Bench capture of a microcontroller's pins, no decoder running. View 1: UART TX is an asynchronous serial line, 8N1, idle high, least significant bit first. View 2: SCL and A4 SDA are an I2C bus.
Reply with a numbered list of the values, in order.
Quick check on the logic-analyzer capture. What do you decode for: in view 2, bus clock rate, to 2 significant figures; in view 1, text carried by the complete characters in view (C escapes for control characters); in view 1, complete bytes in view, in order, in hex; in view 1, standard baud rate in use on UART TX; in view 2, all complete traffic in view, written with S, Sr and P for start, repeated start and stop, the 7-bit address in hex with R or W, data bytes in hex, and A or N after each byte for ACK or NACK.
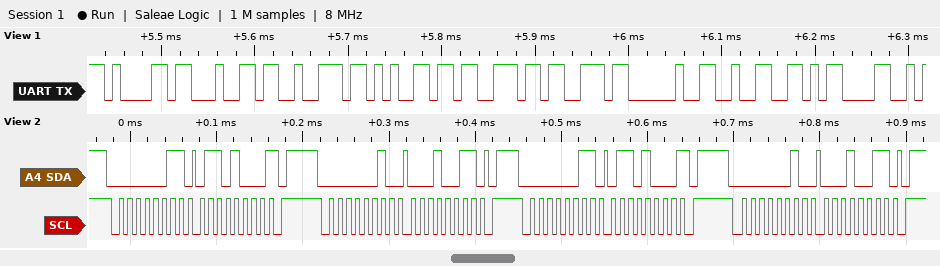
1. 100 kHz
2. "adress 2\r"
3. 61 64 72 65 73 73 20 32 0D
4. 115200 baud
5. S 01R A 68 N P S 01W A 13 A P S 01R A 68 N P S 01W A 13 A P
